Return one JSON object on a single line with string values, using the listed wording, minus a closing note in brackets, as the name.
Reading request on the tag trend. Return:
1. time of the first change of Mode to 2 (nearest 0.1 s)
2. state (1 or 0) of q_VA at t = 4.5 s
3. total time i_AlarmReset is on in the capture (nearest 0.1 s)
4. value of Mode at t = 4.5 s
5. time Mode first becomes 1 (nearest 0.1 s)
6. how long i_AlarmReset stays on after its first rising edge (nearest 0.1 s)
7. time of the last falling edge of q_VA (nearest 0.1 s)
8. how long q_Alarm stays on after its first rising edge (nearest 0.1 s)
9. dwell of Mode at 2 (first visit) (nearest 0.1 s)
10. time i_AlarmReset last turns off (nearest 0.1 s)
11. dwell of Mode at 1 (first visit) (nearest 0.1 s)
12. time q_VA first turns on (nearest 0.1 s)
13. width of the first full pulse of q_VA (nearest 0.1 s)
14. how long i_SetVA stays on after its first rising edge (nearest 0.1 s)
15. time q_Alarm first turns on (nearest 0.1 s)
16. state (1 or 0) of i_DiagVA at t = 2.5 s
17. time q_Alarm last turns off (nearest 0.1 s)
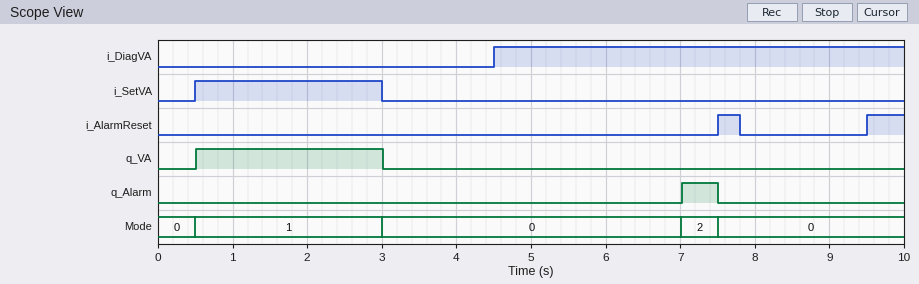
{"time of the first change of Mode to 2": "7.0 s", "state (1 or 0) of q_VA at t = 4.5 s": "0", "total time i_AlarmReset is on in the capture": "0.8 s", "value of Mode at t = 4.5 s": "0", "time Mode first becomes 1": "0.5 s", "how long i_AlarmReset stays on after its first rising edge": "0.3 s", "time of the last falling edge of q_VA": "3.0 s", "how long q_Alarm stays on after its first rising edge": "0.5 s", "dwell of Mode at 2 (first visit)": "0.5 s", "time i_AlarmReset last turns off": "7.8 s", "dwell of Mode at 1 (first visit)": "2.5 s", "time q_VA first turns on": "0.5 s", "width of the first full pulse of q_VA": "2.5 s", "how long i_SetVA stays on after its first rising edge": "2.5 s", "time q_Alarm first turns on": "7.0 s", "state (1 or 0) of i_DiagVA at t = 2.5 s": "0", "time q_Alarm last turns off": "7.5 s"}
